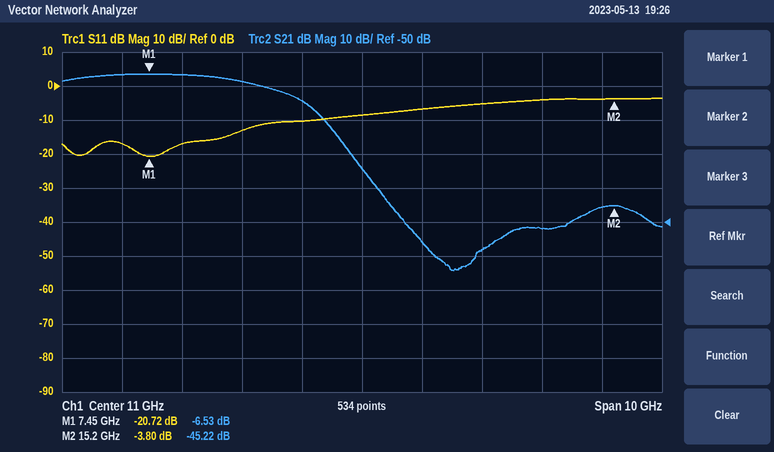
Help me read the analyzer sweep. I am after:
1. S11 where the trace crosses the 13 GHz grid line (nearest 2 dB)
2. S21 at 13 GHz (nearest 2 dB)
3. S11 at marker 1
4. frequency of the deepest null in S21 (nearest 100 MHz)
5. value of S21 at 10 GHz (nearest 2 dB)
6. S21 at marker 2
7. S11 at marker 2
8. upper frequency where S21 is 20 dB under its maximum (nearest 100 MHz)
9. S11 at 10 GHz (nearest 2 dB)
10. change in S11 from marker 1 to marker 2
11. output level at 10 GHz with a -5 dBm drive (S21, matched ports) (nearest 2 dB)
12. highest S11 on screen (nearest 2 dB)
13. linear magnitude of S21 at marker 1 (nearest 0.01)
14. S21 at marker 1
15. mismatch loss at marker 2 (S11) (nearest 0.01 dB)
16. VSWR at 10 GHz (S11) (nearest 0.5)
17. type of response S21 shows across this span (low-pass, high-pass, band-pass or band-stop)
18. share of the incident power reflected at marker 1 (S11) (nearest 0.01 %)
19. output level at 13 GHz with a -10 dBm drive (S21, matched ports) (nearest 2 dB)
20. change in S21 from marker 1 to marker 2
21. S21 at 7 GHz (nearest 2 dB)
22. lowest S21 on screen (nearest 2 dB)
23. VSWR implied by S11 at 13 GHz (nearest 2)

-6 dB
-58 dB
-20.72 dB
12.5 GHz
-14 dB
-45.22 dB
-3.80 dB
10.7 GHz
-10 dB
16.92 dB
-20 dBm
-4 dB
0.47
-6.53 dB
2.34 dB
2.0
low-pass
0.85 %
-68 dBm
-38.69 dB
-6 dB
-64 dB
4
